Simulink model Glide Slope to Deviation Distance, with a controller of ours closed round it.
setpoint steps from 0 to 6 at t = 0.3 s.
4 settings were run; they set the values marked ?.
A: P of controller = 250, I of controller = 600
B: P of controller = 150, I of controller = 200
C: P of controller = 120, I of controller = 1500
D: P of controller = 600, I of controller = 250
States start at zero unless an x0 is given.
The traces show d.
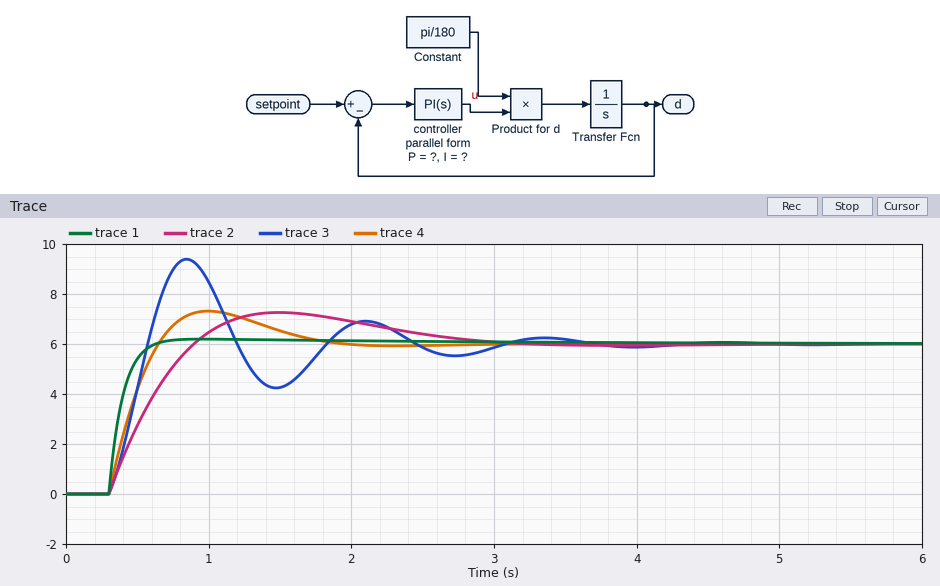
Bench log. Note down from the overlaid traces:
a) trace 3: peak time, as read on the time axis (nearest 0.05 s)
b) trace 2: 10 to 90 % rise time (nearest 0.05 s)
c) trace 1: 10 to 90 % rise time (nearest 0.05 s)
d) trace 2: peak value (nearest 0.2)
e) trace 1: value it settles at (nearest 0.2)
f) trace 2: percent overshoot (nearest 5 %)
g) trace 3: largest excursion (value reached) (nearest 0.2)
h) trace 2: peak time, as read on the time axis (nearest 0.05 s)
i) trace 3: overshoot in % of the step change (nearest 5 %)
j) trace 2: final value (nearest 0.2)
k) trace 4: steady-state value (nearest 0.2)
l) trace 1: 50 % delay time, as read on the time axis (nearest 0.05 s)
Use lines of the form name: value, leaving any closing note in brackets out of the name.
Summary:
trace 3: peak time, as read on the time axis: 0.85 s
trace 2: 10 to 90 % rise time: 0.45 s
trace 1: 10 to 90 % rise time: 0.20 s
trace 2: peak value: 7.2
trace 1: value it settles at: 6.0
trace 2: percent overshoot: 20 %
trace 3: largest excursion (value reached): 9.4
trace 2: peak time, as read on the time axis: 1.50 s
trace 3: overshoot in % of the step change: 55 %
trace 2: final value: 6.0
trace 4: steady-state value: 6.0
trace 1: 50 % delay time, as read on the time axis: 0.35 s
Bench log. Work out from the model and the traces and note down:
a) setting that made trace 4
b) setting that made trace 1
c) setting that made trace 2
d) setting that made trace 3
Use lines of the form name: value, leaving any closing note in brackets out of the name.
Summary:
setting that made trace 4: A
setting that made trace 1: D
setting that made trace 2: B
setting that made trace 3: C
